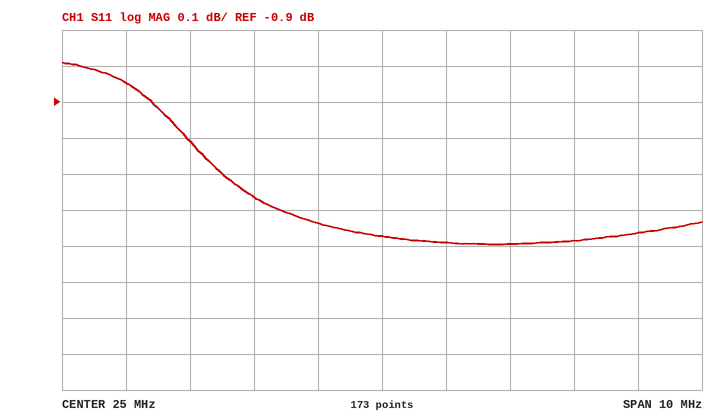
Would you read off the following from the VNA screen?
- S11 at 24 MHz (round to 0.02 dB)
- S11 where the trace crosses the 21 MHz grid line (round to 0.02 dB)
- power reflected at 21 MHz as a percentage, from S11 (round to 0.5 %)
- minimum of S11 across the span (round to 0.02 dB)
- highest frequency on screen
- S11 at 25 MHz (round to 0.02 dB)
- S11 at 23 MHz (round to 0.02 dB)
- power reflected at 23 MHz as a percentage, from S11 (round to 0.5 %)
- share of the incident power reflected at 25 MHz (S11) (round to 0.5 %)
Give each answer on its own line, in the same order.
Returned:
-1.24 dB
-0.84 dB
82.5 %
-1.30 dB
30 MHz
-1.28 dB
-1.16 dB
76.5 %
74.5 %
